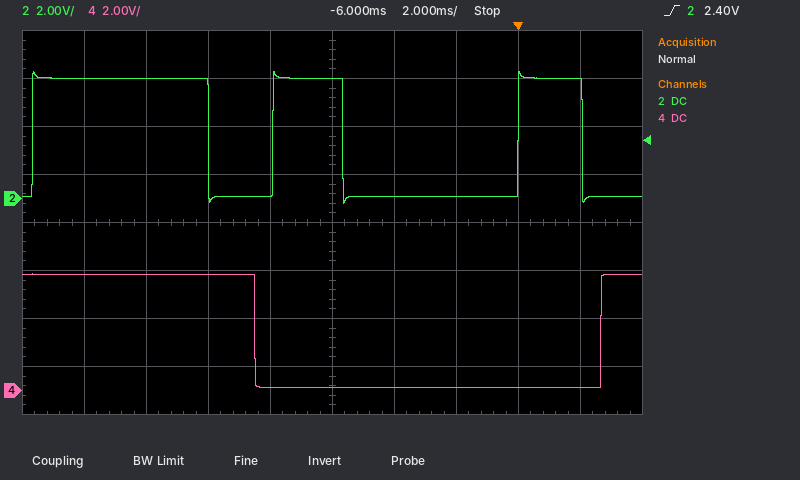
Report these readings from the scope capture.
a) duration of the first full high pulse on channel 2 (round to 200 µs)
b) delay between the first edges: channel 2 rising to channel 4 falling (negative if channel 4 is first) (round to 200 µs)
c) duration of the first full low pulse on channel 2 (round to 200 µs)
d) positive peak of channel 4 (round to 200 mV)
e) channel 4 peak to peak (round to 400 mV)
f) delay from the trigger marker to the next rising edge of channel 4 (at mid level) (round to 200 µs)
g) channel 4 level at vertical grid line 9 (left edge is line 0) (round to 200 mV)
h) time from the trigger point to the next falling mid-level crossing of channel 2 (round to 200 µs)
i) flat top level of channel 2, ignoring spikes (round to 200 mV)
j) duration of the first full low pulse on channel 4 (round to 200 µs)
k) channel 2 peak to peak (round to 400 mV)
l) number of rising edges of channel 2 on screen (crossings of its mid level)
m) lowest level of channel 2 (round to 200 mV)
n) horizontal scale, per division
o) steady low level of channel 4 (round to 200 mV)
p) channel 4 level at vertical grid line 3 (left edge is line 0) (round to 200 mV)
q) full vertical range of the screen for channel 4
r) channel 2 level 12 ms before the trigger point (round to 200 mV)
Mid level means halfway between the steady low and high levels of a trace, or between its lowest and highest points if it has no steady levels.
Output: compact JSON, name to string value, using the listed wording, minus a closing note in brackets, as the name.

{"duration of the first full high pulse on channel 2": "5.6 ms", "delay between the first edges: channel 2 rising to channel 4 falling (negative if channel 4 is first)": "+7.2 ms", "duration of the first full low pulse on channel 2": "2.0 ms", "positive peak of channel 4": "4.8 V", "channel 4 peak to peak": "4.8 V", "delay from the trigger marker to the next rising edge of channel 4 (at mid level)": "2.6 ms", "channel 4 level at vertical grid line 9 (left edge is line 0)": "200 mV", "time from the trigger point to the next falling mid-level crossing of channel 2": "2.0 ms", "flat top level of channel 2, ignoring spikes": "5.0 V", "duration of the first full low pulse on channel 4": "11.2 ms", "channel 2 peak to peak": "5.6 V", "number of rising edges of channel 2 on screen": "3", "lowest level of channel 2": "-200 mV", "horizontal scale, per division": "2 ms", "steady low level of channel 4": "200 mV", "channel 4 level at vertical grid line 3 (left edge is line 0)": "4.8 V", "full vertical range of the screen for channel 4": "16 V", "channel 2 level 12 ms before the trigger point": "5.0 V"}
